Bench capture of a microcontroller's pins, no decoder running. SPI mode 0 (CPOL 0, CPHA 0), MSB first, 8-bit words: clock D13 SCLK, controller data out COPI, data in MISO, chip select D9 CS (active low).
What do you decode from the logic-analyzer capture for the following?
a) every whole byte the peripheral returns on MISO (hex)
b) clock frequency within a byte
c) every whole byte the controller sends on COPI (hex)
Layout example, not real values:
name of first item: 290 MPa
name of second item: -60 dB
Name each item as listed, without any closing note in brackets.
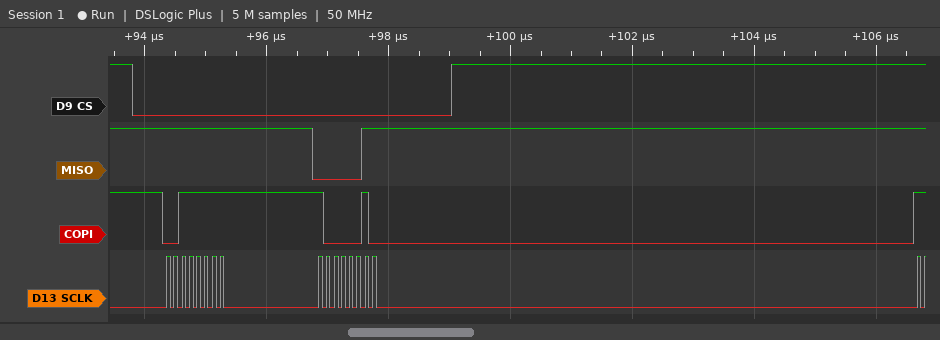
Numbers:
every whole byte the peripheral returns on MISO: FF 03
clock frequency within a byte: 8 MHz
every whole byte the controller sends on COPI: 3F 82
